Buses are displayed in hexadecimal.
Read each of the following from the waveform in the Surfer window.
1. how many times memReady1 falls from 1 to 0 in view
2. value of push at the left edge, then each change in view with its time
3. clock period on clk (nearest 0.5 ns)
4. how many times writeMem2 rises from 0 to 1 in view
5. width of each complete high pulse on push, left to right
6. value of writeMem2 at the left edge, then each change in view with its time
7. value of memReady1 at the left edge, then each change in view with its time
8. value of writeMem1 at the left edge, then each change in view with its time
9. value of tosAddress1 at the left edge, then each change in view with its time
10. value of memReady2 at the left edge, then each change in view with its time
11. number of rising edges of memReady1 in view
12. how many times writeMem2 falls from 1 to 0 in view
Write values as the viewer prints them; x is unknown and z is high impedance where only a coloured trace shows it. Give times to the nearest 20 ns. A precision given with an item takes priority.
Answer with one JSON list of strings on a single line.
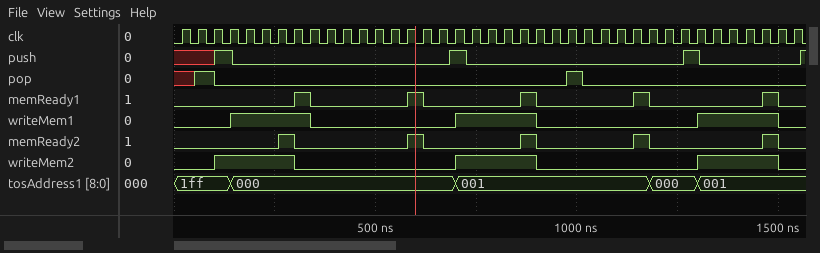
["5", "x, 1 at 100 ns, 0 at 140 ns, 1 at 680 ns, 0 at 720 ns, 1 at 1260 ns, 0 at 1300 ns, 1 at 1560 ns", "40 ns", "3", "40 ns, 40 ns", "0, 1 at 100 ns, 0 at 300 ns, 1 at 700 ns, 0 at 900 ns, 1 at 1300 ns, 0 at 1500 ns", "0, 1 at 300 ns, 0 at 340 ns, 1 at 580 ns, 0 at 620 ns, 1 at 860 ns, 0 at 900 ns, 1 at 1140 ns, 0 at 1180 ns, 1 at 1460 ns, 0 at 1500 ns", "0, 1 at 140 ns, 0 at 340 ns, 1 at 700 ns, 0 at 900 ns, 1 at 1300 ns, 0 at 1500 ns", "1ff, 000 at 140 ns, 001 at 700 ns, 000 at 1180 ns, 001 at 1300 ns", "0, 1 at 260 ns, 0 at 300 ns, 1 at 580 ns, 0 at 620 ns, 1 at 860 ns, 0 at 900 ns, 1 at 1140 ns, 0 at 1180 ns, 1 at 1460 ns, 0 at 1500 ns", "5", "3"]
